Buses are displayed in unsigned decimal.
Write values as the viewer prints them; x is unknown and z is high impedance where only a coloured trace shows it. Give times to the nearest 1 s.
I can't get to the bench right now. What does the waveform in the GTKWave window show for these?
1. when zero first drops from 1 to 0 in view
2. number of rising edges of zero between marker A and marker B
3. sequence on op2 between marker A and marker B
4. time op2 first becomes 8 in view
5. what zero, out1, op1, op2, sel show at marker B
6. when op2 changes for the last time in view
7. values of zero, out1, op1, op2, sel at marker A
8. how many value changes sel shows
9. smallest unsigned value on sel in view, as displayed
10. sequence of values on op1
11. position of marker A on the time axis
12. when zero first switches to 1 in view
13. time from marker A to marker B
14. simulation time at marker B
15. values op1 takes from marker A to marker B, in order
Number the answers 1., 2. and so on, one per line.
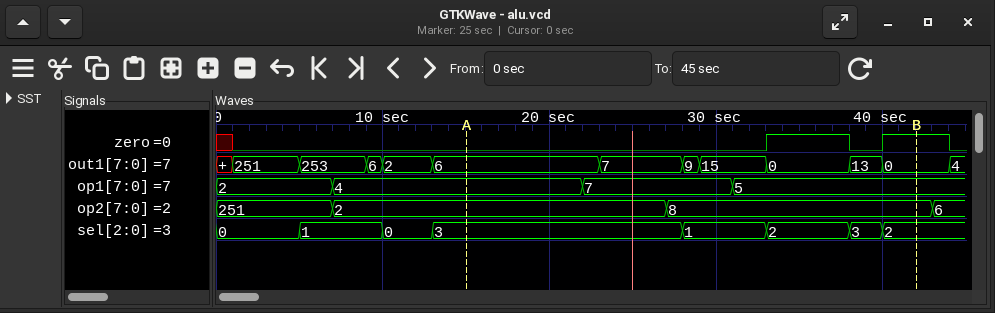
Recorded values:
1. 38 s
2. 2
3. 2, 8
4. 27 s
5. zero=1, out1=0, op1=5, op2=8, sel=2
6. 43 s
7. zero=0, out1=6, op1=4, op2=2, sel=3
8. 7
9. 0
10. 2, 4, 7, 5
11. 15 s
12. 33 s
13. 27 s
14. 42 s
15. 4, 7, 5
